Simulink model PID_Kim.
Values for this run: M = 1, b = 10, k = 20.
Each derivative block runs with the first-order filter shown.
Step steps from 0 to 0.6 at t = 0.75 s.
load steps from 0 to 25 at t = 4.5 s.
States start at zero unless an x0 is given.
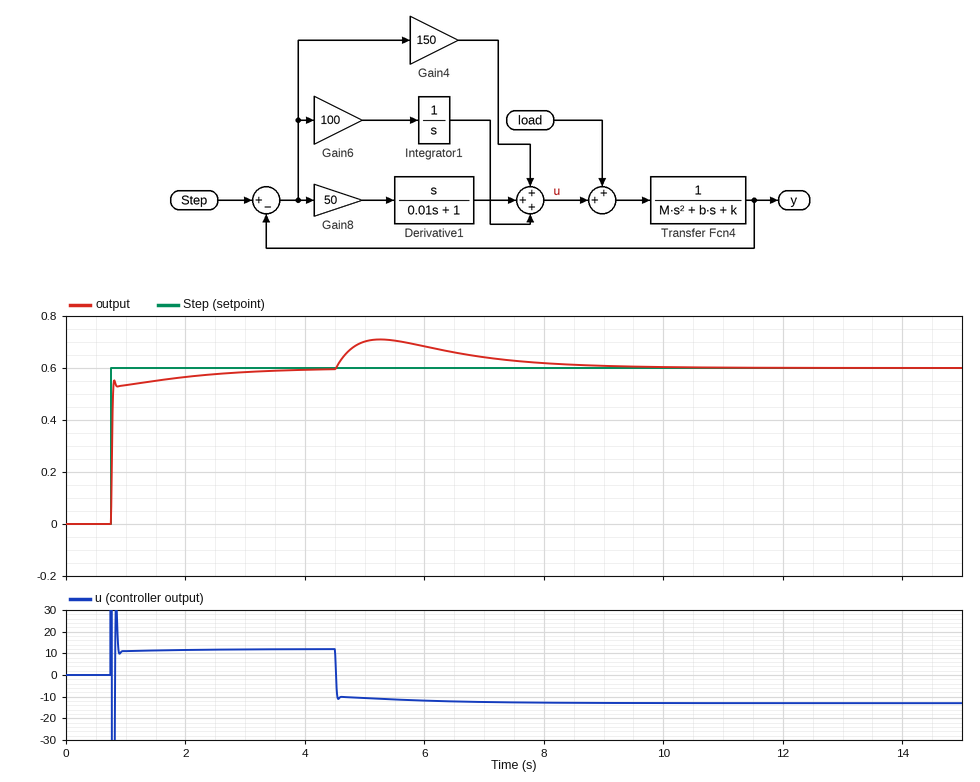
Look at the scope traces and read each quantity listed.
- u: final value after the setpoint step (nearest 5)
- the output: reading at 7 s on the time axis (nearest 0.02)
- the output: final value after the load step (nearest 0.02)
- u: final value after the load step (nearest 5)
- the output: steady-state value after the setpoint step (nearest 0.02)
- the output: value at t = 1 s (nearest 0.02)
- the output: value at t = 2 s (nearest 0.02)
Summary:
10
0.64
0.60
-15
0.60
0.54
0.56
